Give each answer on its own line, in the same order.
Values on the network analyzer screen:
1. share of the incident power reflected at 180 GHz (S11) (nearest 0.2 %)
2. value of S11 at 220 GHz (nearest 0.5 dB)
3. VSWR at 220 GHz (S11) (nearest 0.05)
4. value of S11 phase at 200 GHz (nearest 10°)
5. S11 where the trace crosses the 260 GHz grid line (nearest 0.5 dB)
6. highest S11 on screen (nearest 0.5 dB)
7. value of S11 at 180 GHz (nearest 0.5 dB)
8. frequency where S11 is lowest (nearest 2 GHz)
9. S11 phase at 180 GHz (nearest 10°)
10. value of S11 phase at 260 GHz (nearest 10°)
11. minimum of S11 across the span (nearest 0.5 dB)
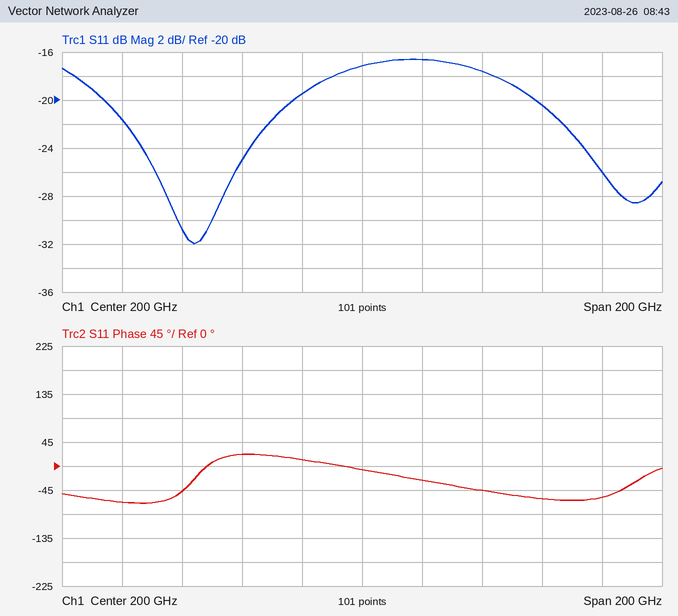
1.2 %
-16.5 dB
1.35
-10°
-20.5 dB
-16.5 dB
-19.5 dB
144 GHz
10°
-60°
-32.0 dB
